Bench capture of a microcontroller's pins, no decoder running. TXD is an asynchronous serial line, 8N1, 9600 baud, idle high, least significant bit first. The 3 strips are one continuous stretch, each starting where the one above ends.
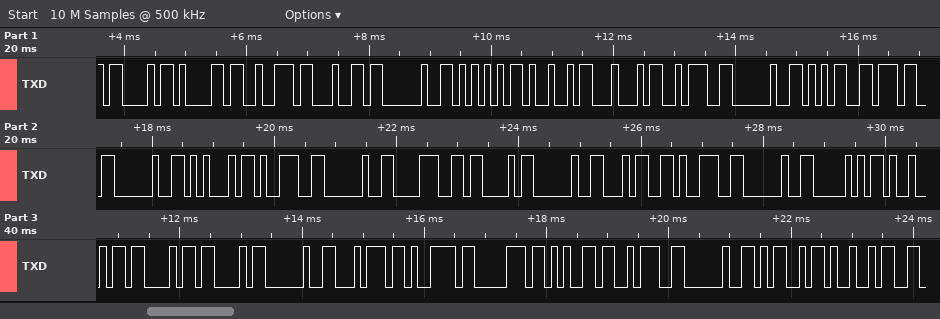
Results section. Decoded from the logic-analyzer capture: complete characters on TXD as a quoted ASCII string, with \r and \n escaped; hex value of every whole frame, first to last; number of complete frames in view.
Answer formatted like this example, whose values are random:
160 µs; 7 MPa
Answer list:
"Card UID: 57 E9 8C 49 PICC type: MI"; 0x43 0x61 0x72 0x64 0x20 0x55 0x49 0x44 0x3A 0x20 0x35 0x37 0x20 0x45 0x39 0x20 0x38 0x43 0x20 0x34 0x39 0x20 0x50 0x49 0x43 0x43 0x20 0x74 0x79 0x70 0x65 0x3A 0x20 0x4D 0x49; 35
